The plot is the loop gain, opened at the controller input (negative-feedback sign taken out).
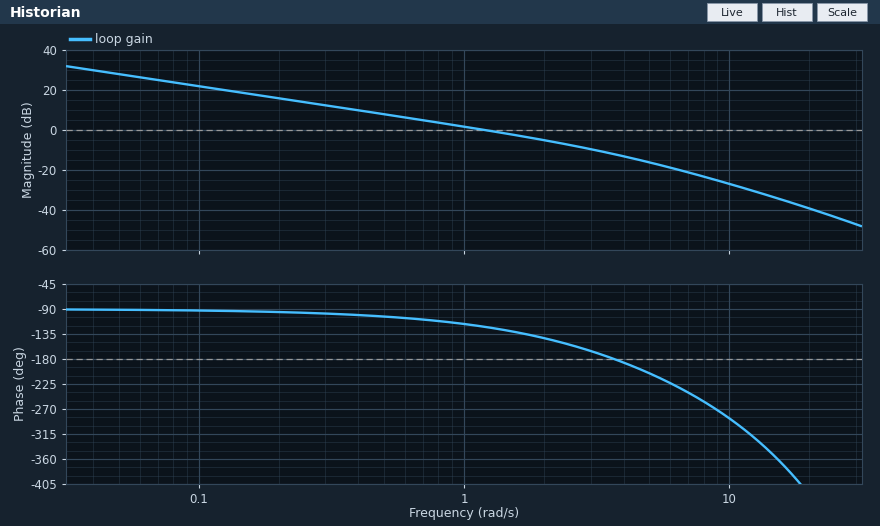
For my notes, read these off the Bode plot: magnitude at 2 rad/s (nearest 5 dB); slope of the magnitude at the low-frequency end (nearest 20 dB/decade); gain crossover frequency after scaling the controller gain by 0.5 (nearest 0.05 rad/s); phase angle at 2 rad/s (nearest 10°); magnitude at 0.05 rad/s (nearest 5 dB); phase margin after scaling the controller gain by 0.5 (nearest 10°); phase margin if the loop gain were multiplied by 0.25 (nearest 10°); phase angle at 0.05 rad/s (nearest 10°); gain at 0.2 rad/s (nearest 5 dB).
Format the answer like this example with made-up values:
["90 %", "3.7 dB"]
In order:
["-5 dB", "-20 dB/decade", "0.60 rad/s", "-140°", "30 dB", "70°", "80°", "-90°", "15 dB"]
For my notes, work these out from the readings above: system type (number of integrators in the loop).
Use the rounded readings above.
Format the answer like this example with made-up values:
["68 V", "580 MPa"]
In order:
["1"]
